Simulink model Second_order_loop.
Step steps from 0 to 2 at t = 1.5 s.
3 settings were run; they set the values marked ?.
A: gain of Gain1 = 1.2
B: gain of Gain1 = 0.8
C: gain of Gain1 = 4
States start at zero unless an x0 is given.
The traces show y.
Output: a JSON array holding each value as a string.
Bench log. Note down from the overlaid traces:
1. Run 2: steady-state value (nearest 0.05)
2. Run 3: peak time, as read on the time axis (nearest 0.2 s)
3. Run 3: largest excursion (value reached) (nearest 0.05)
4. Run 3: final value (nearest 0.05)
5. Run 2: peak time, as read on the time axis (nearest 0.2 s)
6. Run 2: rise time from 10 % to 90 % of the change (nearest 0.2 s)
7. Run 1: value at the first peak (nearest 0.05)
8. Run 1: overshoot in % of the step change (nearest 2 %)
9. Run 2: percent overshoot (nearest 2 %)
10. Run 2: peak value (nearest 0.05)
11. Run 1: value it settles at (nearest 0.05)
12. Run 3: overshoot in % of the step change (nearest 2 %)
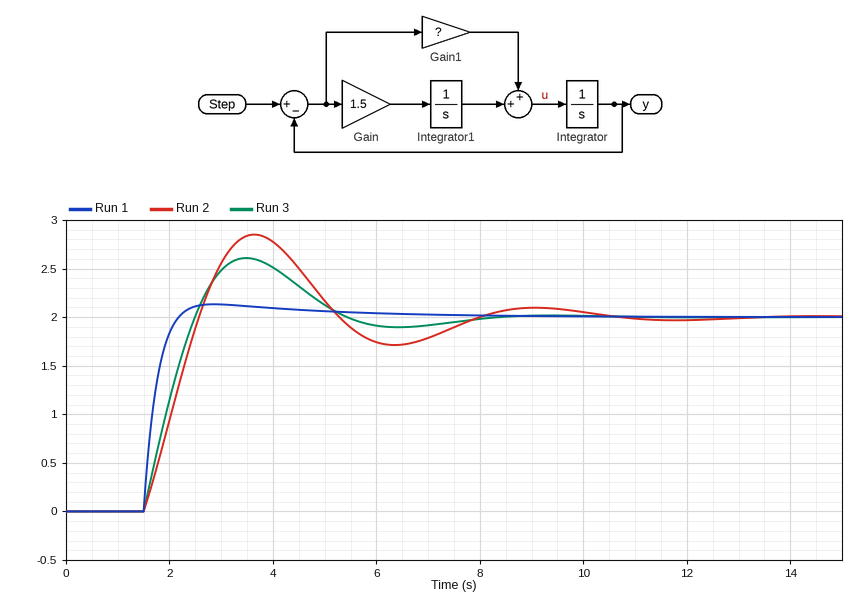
["2.00", "3.4 s", "2.60", "2.00", "3.6 s", "0.8 s", "2.15", "6 %", "42 %", "2.85", "2.00", "30 %"]
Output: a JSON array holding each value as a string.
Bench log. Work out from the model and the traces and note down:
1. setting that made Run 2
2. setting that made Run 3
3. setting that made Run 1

["B", "A", "C"]
